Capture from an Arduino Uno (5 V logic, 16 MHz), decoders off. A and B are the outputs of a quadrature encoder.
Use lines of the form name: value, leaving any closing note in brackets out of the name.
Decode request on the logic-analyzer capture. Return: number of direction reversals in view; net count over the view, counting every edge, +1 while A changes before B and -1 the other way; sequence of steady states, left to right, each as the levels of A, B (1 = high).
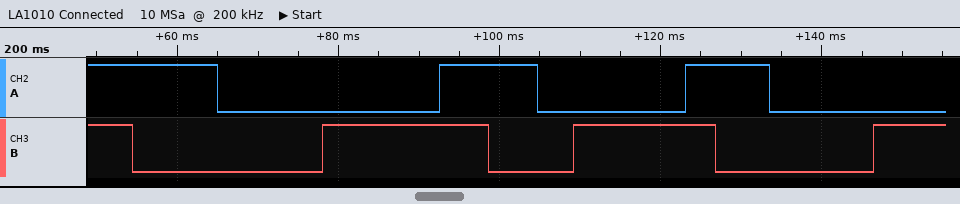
number of direction reversals in view: 0
net count over the view, counting every edge, +1 while A changes before B and -1 the other way: -11
sequence of steady states, left to right, each as the levels of A, B: 11 10 00 01 11 10 00 01 11 10 00 01
